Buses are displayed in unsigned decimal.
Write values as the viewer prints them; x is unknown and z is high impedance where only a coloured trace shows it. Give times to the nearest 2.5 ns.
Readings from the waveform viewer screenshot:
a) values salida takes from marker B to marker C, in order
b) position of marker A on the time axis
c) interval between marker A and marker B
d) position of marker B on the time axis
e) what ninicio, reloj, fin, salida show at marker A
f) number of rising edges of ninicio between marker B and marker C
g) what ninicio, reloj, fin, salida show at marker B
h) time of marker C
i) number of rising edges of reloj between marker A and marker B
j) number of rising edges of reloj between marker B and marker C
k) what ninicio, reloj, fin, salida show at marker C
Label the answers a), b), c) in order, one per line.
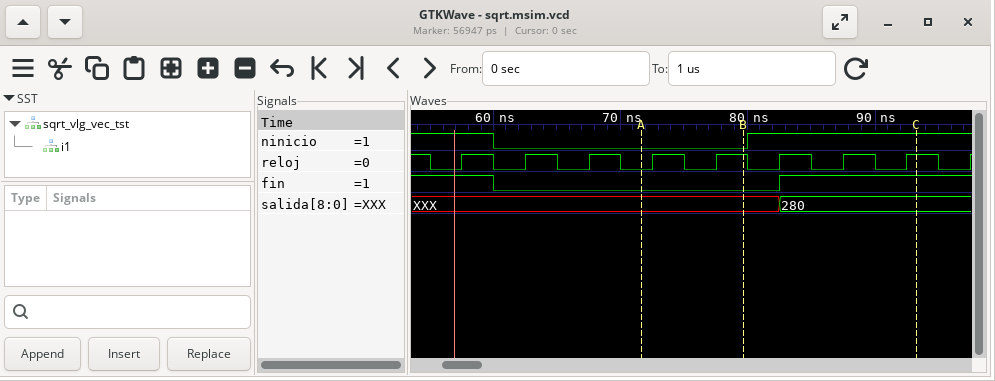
a) XXX, 280
b) 72.5 ns
c) 7.5 ns
d) 80 ns
e) ninicio=0, reloj=0, fin=0, salida=XXX
f) 1
g) ninicio=0, reloj=1, fin=0, salida=XXX
h) 92.5 ns
i) 2
j) 3
k) ninicio=1, reloj=1, fin=1, salida=280
